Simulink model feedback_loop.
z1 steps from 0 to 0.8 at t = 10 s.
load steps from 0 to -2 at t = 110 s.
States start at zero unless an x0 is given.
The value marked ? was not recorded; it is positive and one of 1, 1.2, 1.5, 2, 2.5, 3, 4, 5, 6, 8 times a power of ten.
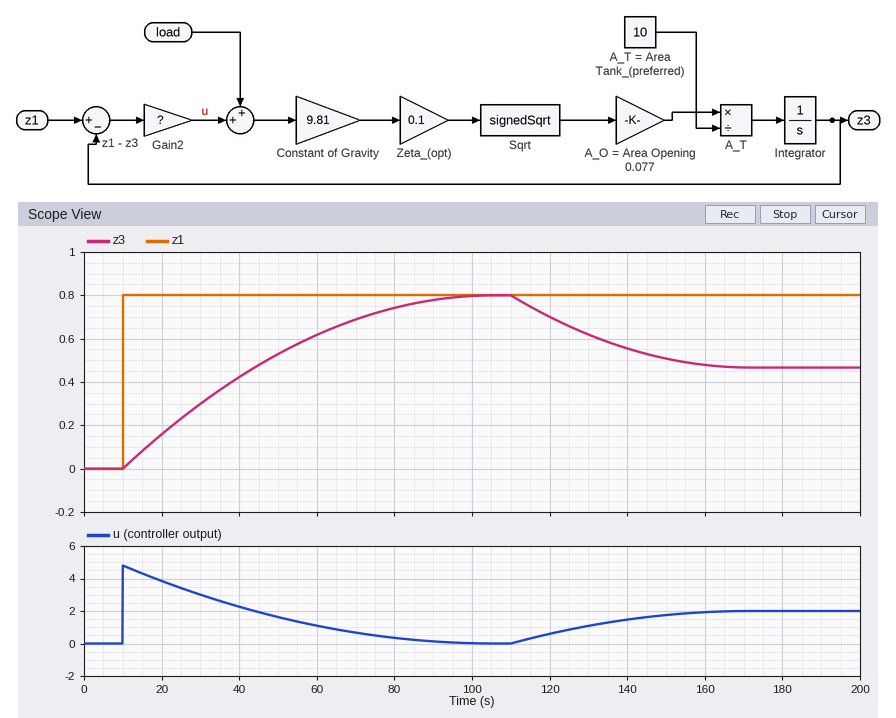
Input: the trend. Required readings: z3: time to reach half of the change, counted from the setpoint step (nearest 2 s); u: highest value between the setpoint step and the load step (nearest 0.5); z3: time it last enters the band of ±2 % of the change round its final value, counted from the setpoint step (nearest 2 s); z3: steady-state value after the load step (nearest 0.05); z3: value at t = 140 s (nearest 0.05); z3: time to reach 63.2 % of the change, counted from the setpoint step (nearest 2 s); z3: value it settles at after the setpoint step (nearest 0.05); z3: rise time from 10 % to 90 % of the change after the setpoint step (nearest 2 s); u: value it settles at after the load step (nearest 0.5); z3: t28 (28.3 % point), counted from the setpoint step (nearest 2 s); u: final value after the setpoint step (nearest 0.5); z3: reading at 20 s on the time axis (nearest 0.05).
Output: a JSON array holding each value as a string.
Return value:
["28 s", "5.0", "82 s", "0.45", "0.55", "38 s", "0.80", "60 s", "2.0", "14 s", "0.0", "0.15"]
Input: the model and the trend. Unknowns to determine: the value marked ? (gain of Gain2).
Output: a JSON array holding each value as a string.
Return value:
["6"]
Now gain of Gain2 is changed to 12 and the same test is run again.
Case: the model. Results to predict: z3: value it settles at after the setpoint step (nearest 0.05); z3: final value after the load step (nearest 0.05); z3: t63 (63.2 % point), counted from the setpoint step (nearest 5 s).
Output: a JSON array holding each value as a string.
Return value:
["0.80", "0.65", "25 s"]
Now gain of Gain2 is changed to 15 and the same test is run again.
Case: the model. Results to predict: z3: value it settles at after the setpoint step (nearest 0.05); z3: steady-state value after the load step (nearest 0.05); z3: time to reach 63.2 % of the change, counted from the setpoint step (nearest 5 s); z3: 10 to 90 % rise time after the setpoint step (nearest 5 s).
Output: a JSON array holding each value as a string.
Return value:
["0.80", "0.65", "25 s", "40 s"]
